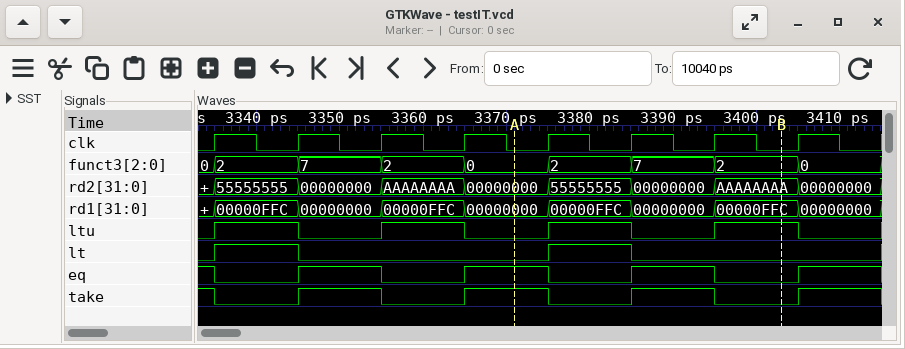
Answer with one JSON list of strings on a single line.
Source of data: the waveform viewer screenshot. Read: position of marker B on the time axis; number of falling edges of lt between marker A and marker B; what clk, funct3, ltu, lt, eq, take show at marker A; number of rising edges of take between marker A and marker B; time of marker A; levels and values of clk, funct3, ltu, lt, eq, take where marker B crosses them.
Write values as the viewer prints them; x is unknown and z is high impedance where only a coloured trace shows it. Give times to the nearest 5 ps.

["3405 ps", "1", "clk=0, funct3=0, ltu=0, lt=0, eq=1, take=1", "1", "3370 ps", "clk=0, funct3=2, ltu=1, lt=0, eq=0, take=0"]
